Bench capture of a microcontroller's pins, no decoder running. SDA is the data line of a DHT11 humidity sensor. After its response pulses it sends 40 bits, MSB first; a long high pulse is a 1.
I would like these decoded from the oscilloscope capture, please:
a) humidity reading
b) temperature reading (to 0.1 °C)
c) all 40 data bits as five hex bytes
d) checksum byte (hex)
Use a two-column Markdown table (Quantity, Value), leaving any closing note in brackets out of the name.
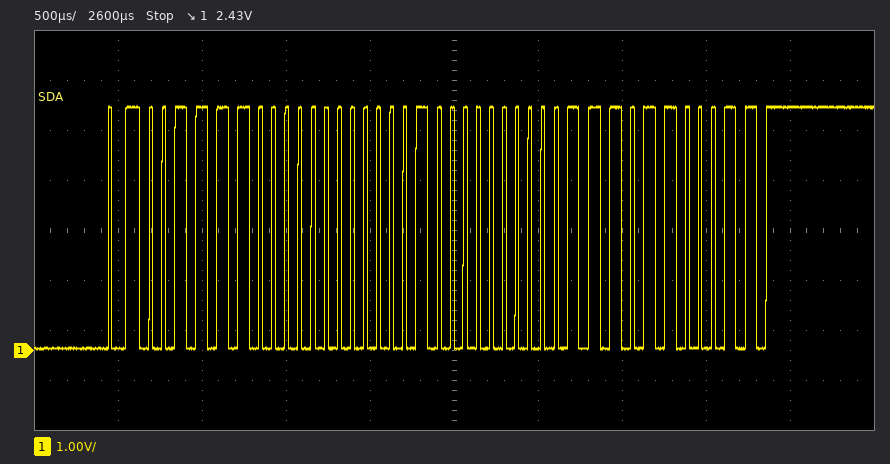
| Quantity | Value |
|---|---|
| humidity reading | 60 % |
| temperature reading | 32.7 °C |
| all 40 data bits as five hex bytes | 3C 00 20 07 63 |
| checksum byte | 0x63 |
